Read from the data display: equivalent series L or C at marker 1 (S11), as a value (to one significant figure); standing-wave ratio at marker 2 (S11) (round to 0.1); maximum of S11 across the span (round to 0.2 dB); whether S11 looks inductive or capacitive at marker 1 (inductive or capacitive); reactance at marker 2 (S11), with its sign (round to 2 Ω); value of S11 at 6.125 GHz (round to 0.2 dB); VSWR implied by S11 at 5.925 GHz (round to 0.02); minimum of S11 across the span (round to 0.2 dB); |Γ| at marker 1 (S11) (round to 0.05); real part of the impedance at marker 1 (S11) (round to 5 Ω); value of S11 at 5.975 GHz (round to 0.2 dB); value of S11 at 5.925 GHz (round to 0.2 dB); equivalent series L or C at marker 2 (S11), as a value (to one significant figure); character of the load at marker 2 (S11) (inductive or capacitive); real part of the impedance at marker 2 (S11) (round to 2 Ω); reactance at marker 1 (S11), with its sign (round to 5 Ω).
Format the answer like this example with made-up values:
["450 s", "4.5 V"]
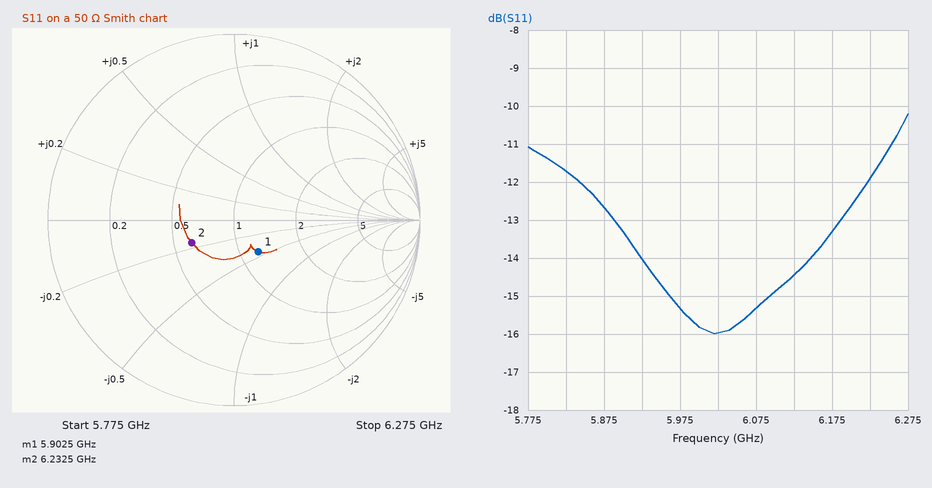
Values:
["1 pF", "1.7", "-10.2 dB", "capacitive", "-8 Ω", "-14.4 dB", "1.50", "-16.0 dB", "0.20", "60 Ω", "-15.4 dB", "-14.0 dB", "3 pF", "capacitive", "30 Ω", "-20 Ω"]
